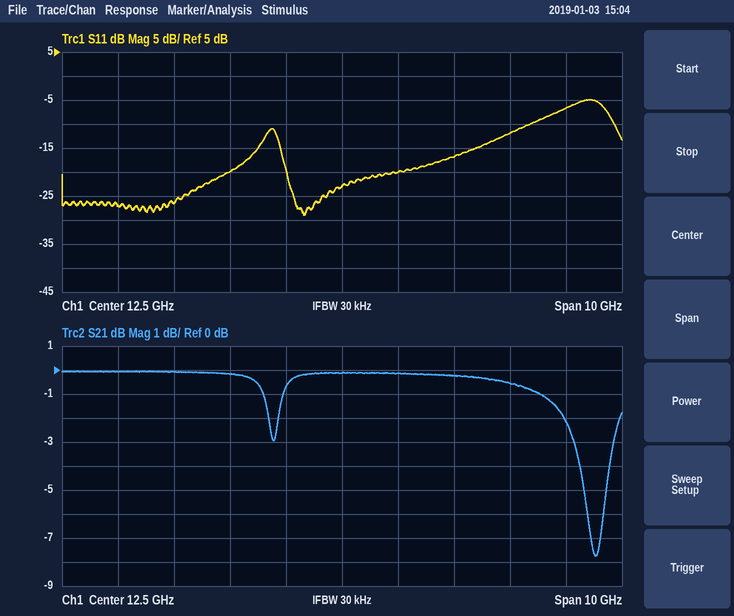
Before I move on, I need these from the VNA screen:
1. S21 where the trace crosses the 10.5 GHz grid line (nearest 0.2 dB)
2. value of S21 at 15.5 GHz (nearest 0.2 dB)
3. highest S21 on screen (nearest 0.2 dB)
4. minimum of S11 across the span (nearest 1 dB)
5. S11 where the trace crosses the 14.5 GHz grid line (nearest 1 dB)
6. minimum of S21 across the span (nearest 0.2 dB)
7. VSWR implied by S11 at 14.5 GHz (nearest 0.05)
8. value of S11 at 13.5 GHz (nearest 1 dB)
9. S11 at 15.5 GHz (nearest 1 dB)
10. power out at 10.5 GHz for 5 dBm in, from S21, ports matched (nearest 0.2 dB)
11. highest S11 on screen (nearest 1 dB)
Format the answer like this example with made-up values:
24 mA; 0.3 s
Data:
-0.2 dB; -0.6 dB; 0.0 dB; -29 dB; -17 dB; -7.8 dB; 1.35; -20 dB; -12 dB; 4.8 dBm; -5 dB
